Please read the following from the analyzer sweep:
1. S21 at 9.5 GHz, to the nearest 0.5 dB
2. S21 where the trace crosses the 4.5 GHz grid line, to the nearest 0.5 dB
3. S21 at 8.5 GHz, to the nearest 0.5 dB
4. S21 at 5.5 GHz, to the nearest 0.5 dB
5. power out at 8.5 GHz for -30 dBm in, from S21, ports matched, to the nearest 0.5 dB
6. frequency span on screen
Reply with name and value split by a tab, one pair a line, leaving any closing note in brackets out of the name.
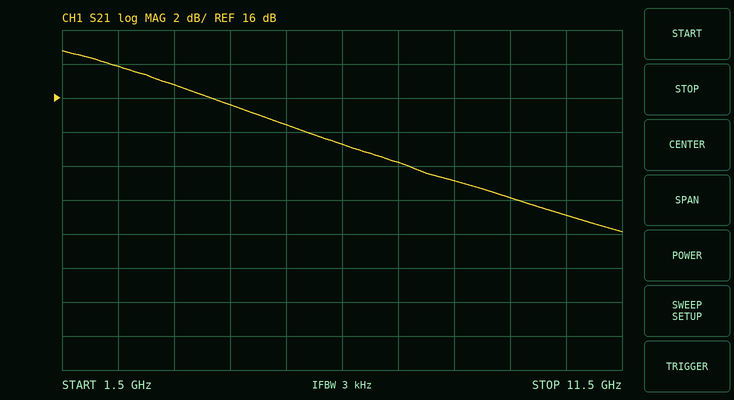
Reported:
S21 at 9.5 GHz, to the nearest 0.5 dB	10.0 dB
S21 where the trace crosses the 4.5 GHz grid line, to the nearest 0.5 dB	15.5 dB
S21 at 8.5 GHz, to the nearest 0.5 dB	11.0 dB
S21 at 5.5 GHz, to the nearest 0.5 dB	14.5 dB
power out at 8.5 GHz for -30 dBm in, from S21, ports matched, to the nearest 0.5 dB	-19.0 dBm
frequency span on screen	10 GHz
